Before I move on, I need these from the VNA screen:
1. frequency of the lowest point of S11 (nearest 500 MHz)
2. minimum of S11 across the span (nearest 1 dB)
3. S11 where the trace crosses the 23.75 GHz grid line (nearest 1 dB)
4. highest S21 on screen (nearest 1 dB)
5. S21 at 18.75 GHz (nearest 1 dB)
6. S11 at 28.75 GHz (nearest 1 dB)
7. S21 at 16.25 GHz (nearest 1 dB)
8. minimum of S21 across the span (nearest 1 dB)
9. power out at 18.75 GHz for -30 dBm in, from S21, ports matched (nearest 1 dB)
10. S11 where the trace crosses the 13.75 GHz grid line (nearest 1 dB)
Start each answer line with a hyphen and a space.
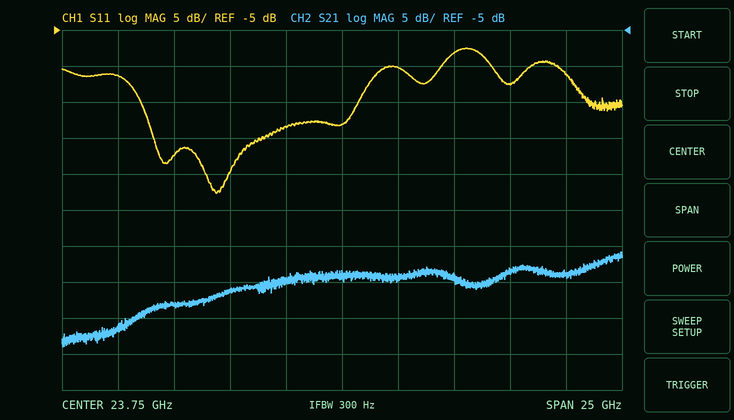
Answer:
- 18.0 GHz
- -28 dB
- -18 dB
- -36 dB
- -41 dB
- -8 dB
- -43 dB
- -49 dB
- -71 dBm
- -11 dB
